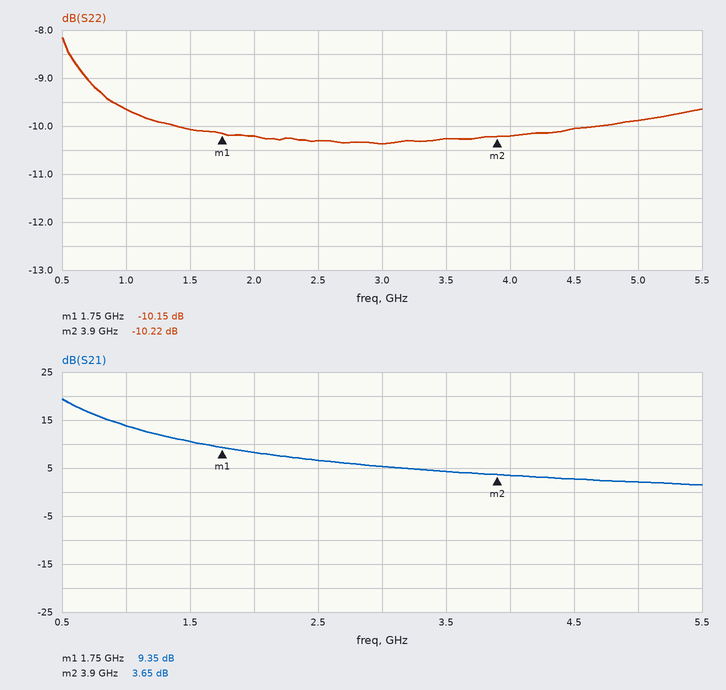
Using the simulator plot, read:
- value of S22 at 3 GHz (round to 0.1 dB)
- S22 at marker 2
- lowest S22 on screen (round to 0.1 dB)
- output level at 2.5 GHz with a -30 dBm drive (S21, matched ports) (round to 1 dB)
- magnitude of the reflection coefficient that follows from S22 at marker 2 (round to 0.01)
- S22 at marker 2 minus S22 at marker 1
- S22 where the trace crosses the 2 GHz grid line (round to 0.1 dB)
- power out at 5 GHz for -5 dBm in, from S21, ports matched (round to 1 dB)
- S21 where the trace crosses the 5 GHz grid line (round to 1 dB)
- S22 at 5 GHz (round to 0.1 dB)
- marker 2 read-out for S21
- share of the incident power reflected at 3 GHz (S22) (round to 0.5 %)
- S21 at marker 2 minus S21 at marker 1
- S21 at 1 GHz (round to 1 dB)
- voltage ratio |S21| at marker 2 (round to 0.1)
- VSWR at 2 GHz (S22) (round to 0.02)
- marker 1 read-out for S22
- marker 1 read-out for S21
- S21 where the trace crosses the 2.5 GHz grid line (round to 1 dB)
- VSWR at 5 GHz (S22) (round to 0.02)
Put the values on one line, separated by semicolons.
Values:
-10.4 dB; -10.22 dB; -10.4 dB; -23 dBm; 0.31; -0.07 dB; -10.2 dB; -3 dBm; 2 dB; -9.9 dB; 3.65 dB; 9.0 %; -5.70 dB; 14 dB; 1.5; 1.90; -10.15 dB; 9.35 dB; 7 dB; 1.94
